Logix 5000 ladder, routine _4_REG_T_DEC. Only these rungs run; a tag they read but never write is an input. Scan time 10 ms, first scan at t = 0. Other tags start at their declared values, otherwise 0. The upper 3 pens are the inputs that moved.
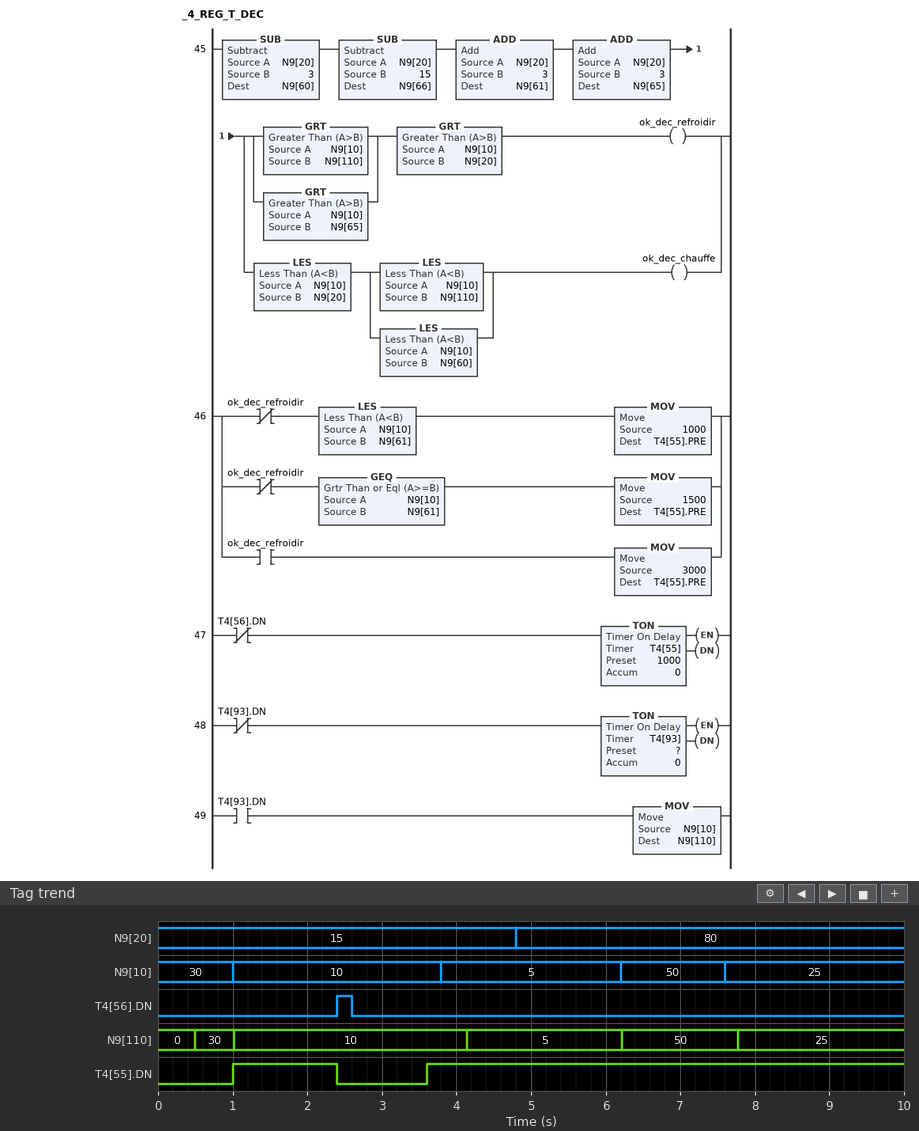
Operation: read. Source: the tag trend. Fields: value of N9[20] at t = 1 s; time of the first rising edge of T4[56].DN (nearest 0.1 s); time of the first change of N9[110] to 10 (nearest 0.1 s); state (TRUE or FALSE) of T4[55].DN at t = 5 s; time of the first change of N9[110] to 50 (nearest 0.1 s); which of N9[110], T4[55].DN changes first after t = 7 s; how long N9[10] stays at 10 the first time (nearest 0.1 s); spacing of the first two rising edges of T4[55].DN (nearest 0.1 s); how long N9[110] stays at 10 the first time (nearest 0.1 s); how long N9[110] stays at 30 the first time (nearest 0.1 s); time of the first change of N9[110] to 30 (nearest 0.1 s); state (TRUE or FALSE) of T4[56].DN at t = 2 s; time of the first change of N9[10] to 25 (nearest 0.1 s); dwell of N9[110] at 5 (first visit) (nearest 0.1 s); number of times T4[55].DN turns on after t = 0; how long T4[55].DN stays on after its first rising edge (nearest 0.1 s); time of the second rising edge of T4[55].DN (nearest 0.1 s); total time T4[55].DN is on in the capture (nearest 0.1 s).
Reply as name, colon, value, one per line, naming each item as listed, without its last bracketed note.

value of N9[20] at t = 1 s: 15
time of the first rising edge of T4[56].DN: 2.4 s
time of the first change of N9[110] to 10: 1.0 s
state (TRUE or FALSE) of T4[55].DN at t = 5 s: TRUE
time of the first change of N9[110] to 50: 6.2 s
which of N9[110], T4[55].DN changes first after t = 7 s: N9[110]
how long N9[10] stays at 10 the first time: 2.8 s
spacing of the first two rising edges of T4[55].DN: 2.6 s
how long N9[110] stays at 10 the first time: 3.1 s
how long N9[110] stays at 30 the first time: 0.5 s
time of the first change of N9[110] to 30: 0.5 s
state (TRUE or FALSE) of T4[56].DN at t = 2 s: FALSE
time of the first change of N9[10] to 25: 7.6 s
dwell of N9[110] at 5 (first visit): 2.1 s
number of times T4[55].DN turns on after t = 0: 2
how long T4[55].DN stays on after its first rising edge: 1.4 s
time of the second rising edge of T4[55].DN: 3.6 s
total time T4[55].DN is on in the capture: 7.8 s
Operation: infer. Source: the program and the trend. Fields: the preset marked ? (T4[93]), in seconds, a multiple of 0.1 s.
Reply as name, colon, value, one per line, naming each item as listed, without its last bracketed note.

the preset marked ? (T4[93]), in seconds, a multiple of 0.1 s: 0.5 s
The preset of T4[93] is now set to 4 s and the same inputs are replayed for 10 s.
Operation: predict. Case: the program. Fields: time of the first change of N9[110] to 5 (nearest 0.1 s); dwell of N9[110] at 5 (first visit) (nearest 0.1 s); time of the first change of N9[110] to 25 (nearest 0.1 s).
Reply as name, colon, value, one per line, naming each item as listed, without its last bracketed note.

time of the first change of N9[110] to 5: 4.0 s
dwell of N9[110] at 5 (first visit): 4.0 s
time of the first change of N9[110] to 25: 8.0 s
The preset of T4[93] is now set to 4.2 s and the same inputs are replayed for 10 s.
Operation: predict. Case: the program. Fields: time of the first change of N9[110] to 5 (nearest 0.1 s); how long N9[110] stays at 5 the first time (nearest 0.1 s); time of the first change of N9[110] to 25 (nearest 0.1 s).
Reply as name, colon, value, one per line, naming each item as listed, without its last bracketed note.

time of the first change of N9[110] to 5: 4.2 s
how long N9[110] stays at 5 the first time: 4.2 s
time of the first change of N9[110] to 25: 8.4 s
